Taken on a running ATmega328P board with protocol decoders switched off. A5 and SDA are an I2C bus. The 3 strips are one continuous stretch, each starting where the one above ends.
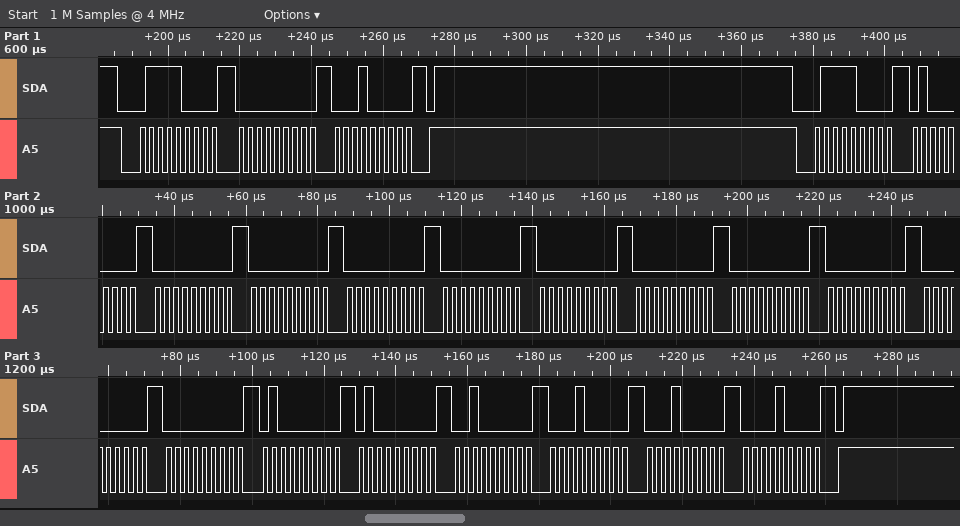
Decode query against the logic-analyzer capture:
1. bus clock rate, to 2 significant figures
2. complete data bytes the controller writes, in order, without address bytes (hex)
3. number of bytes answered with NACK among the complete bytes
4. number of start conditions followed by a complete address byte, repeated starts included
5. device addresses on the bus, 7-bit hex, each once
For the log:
400 kHz
00 10 40 00 00 00 00 00 00 00 00 00 00 40 40 20 10 10 08
0
2
0x3C
